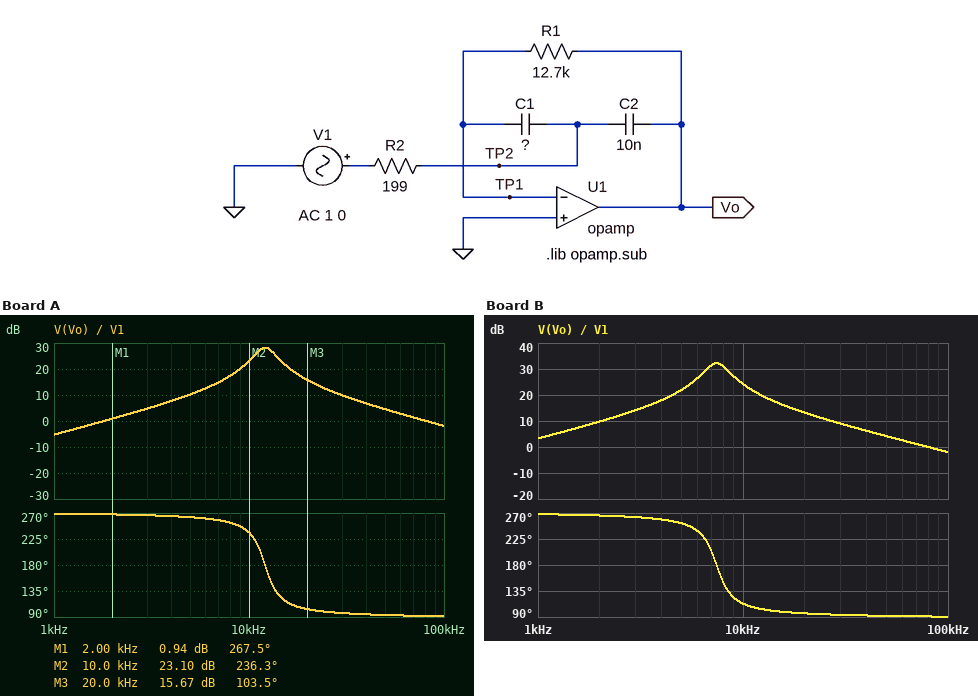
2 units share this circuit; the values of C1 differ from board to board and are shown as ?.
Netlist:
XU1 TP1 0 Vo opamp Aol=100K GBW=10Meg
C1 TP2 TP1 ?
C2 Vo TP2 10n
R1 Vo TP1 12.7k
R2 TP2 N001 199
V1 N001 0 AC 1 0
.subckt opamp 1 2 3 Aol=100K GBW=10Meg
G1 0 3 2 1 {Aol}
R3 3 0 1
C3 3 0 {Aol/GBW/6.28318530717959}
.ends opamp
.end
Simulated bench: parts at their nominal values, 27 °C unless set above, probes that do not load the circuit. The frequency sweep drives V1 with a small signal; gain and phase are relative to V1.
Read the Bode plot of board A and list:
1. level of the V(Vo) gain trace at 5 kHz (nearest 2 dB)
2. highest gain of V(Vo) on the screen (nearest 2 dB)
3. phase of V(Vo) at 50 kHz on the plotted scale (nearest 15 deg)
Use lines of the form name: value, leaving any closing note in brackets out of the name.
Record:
level of the V(Vo) gain trace at 5 kHz: 10 dB
highest gain of V(Vo) on the screen: 28 dB
phase of V(Vo) at 50 kHz on the plotted scale: 90 deg
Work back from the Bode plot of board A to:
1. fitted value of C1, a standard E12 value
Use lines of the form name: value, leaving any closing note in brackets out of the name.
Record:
fitted value of C1, a standard E12 value: 6.8 nF
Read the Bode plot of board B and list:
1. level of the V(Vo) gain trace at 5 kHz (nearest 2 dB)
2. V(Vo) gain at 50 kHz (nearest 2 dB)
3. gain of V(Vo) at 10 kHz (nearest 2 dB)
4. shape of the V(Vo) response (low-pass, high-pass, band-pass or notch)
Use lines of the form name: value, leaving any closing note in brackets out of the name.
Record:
level of the V(Vo) gain trace at 5 kHz: 22 dB
V(Vo) gain at 50 kHz: 4 dB
gain of V(Vo) at 10 kHz: 24 dB
shape of the V(Vo) response: band-pass
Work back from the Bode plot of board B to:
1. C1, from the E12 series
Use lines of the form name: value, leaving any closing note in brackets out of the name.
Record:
C1, from the E12 series: 18 nF
